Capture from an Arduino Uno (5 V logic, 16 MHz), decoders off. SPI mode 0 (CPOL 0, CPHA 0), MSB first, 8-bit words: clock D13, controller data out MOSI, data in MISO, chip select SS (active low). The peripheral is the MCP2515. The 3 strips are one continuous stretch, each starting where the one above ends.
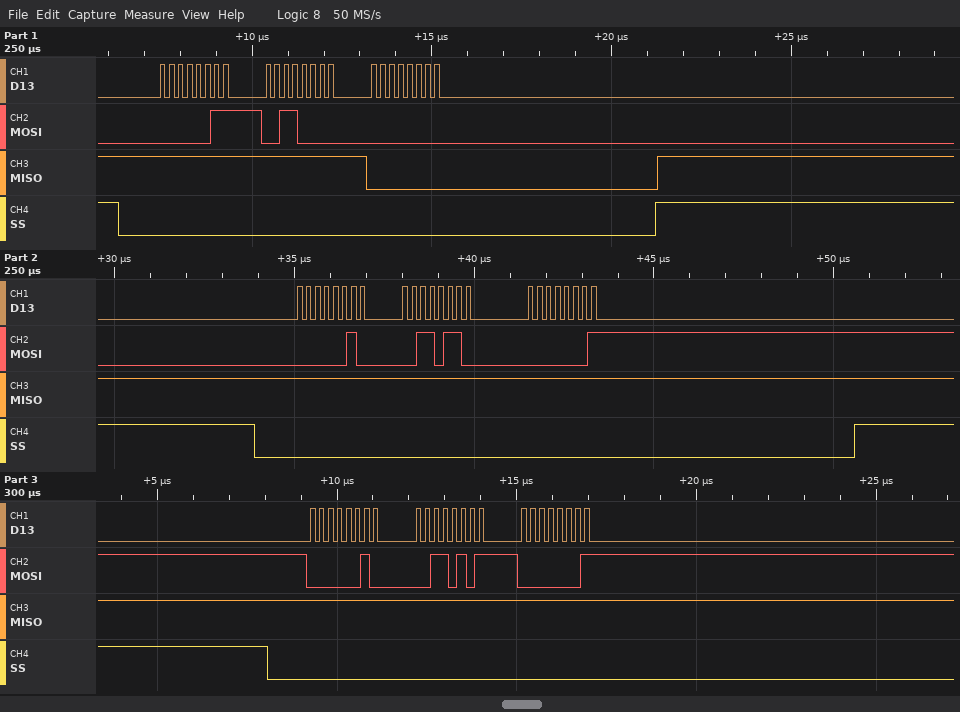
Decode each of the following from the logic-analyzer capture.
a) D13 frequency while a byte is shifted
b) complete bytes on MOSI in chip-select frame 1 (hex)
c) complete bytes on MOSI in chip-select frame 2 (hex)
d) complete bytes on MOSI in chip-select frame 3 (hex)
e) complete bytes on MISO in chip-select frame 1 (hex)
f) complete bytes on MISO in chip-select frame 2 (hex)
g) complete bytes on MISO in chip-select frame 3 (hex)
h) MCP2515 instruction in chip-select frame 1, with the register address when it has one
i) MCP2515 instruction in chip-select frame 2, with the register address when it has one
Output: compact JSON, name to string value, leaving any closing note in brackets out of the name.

{"D13 frequency while a byte is shifted": "4 MHz", "complete bytes on MOSI in chip-select frame 1": "03 30 00", "complete bytes on MOSI in chip-select frame 2": "02 36 01", "complete bytes on MOSI in chip-select frame 3": "02 35 01", "complete bytes on MISO in chip-select frame 1": "FF FF 00", "complete bytes on MISO in chip-select frame 2": "FF FF FF", "complete bytes on MISO in chip-select frame 3": "FF FF FF", "MCP2515 instruction in chip-select frame 1, with the register address when it has one": "READ 0x30", "MCP2515 instruction in chip-select frame 2, with the register address when it has one": "WRITE 0x36"}
